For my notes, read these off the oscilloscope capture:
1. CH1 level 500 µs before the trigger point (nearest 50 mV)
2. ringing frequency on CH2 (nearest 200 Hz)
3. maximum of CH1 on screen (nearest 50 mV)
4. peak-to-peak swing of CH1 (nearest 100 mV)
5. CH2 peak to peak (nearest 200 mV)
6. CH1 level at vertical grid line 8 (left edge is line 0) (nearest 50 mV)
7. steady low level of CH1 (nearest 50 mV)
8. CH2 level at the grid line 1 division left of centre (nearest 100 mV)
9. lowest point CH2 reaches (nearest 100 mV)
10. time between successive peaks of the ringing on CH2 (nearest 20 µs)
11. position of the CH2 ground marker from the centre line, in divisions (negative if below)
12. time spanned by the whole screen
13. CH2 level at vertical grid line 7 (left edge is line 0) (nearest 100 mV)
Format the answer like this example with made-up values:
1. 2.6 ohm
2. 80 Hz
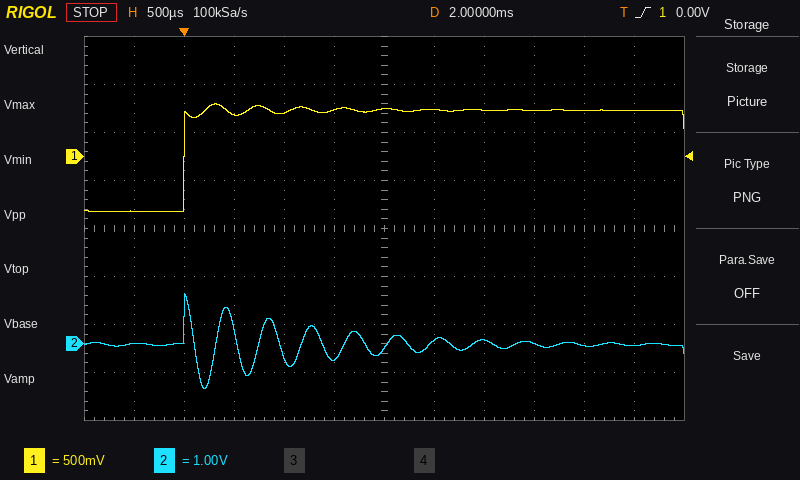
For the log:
1. -550 mV
2. 2.4 kHz
3. 550 mV
4. 1.10 V
5. 2.0 V
6. 500 mV
7. -550 mV
8. -300 mV
9. -900 mV
10. 420 µs
11. -2.4 div
12. 6 ms
13. 100 mV
